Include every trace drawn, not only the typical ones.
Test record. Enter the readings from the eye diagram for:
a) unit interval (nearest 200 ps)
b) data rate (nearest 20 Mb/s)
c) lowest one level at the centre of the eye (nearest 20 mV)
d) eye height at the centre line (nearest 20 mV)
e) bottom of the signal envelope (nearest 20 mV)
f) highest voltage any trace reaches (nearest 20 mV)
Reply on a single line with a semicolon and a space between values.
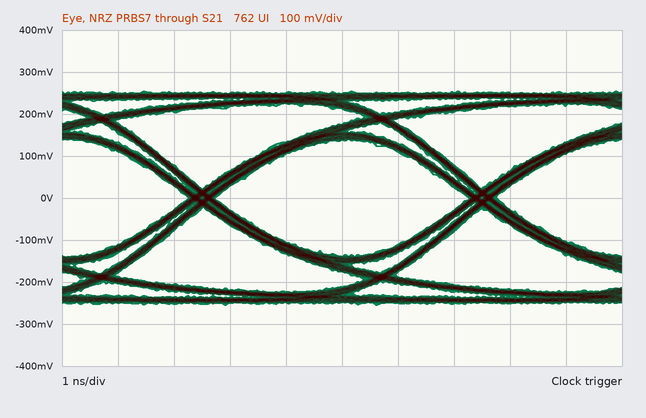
5.0 ns; 200 Mb/s; 140 mV; 280 mV; -260 mV; 260 mV
